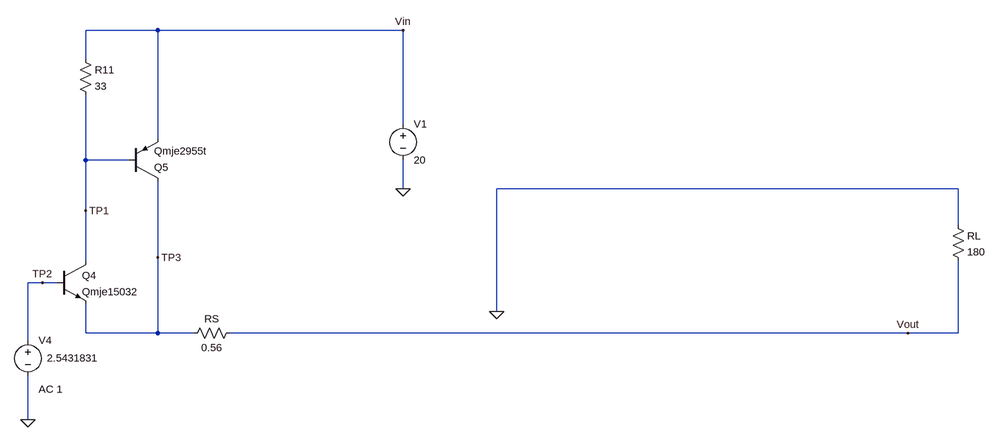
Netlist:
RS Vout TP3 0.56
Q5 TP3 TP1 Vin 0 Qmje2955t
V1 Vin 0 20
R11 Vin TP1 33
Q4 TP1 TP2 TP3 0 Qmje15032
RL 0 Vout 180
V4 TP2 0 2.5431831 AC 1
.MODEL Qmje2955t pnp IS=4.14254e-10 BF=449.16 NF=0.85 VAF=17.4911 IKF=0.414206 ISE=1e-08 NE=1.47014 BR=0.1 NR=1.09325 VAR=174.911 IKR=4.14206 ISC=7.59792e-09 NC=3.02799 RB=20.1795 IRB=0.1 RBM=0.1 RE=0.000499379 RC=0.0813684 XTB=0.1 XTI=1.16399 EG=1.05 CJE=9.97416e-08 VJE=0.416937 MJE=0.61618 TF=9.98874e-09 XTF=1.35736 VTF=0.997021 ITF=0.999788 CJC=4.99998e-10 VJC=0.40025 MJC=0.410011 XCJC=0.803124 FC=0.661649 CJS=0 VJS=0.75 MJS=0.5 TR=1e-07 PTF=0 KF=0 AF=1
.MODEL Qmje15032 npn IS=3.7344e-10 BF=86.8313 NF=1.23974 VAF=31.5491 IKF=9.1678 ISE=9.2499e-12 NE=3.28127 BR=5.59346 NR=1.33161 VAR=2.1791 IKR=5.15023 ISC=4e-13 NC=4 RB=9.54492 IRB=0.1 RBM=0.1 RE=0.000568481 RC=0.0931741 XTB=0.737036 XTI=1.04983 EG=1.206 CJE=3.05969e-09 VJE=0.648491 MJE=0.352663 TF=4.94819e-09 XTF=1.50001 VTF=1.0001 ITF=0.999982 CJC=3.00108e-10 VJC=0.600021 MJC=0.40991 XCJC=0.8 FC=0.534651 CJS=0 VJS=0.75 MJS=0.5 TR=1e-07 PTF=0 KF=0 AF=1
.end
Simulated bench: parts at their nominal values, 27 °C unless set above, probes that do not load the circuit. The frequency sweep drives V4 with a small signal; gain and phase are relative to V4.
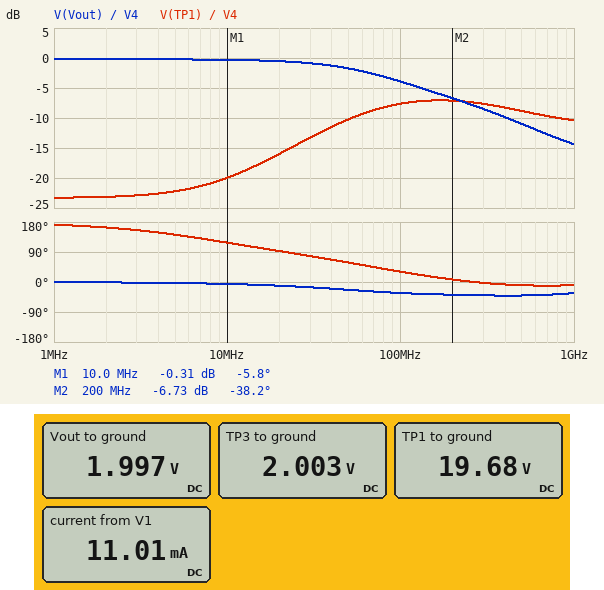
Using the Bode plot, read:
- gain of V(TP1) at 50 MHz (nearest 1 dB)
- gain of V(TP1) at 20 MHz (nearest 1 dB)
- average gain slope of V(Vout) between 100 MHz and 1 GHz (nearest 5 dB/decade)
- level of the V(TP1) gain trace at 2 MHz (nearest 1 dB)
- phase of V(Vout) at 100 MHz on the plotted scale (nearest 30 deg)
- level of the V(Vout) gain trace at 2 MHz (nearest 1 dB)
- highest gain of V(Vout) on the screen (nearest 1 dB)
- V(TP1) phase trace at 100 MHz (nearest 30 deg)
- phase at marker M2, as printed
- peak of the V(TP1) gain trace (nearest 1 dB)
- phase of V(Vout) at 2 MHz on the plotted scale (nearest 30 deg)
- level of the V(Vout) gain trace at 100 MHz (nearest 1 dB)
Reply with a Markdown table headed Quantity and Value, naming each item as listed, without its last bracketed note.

| Quantity | Value |
|---|---|
| gain of V(TP1) at 50 MHz | -10 dB |
| gain of V(TP1) at 20 MHz | -16 dB |
| average gain slope of V(Vout) between 100 MHz and 1 GHz | -10 dB/decade |
| level of the V(TP1) gain trace at 2 MHz | -23 dB |
| phase of V(Vout) at 100 MHz on the plotted scale | -30 deg |
| level of the V(Vout) gain trace at 2 MHz | 0 dB |
| highest gain of V(Vout) on the screen | 0 dB |
| V(TP1) phase trace at 100 MHz | 30 deg |
| phase at marker M2, as printed | -38.2 deg |
| peak of the V(TP1) gain trace | -7 dB |
| phase of V(Vout) at 2 MHz on the plotted scale | 0 deg |
| level of the V(Vout) gain trace at 100 MHz | -4 dB |
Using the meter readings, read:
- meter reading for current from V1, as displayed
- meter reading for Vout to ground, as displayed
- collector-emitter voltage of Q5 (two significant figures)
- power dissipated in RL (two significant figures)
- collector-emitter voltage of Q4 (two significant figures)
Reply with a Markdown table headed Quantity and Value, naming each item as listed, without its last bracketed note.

| Quantity | Value |
|---|---|
| meter reading for current from V1, as displayed | 11.01 mA |
| meter reading for Vout to ground, as displayed | 1.997 V |
| collector-emitter voltage of Q5 | -18 V |
| power dissipated in RL | 22 mW |
| collector-emitter voltage of Q4 | 18 V |
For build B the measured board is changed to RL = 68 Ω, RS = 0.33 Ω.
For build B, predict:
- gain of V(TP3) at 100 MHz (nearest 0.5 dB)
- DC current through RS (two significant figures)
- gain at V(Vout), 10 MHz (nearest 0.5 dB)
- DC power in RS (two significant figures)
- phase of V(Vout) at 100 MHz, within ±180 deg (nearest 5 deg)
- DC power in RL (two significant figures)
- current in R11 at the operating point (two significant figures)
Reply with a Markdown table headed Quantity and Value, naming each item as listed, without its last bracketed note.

| Quantity | Value |
|---|---|
| gain of V(TP3) at 100 MHz | -4.5 dB |
| DC current through RS | 29 mA |
| gain at V(Vout), 10 MHz | -1.0 dB |
| DC power in RS | 280 µW |
| phase of V(Vout) at 100 MHz, within ±180 deg | -30 deg |
| DC power in RL | 58 mW |
| current in R11 at the operating point | 11 mA |
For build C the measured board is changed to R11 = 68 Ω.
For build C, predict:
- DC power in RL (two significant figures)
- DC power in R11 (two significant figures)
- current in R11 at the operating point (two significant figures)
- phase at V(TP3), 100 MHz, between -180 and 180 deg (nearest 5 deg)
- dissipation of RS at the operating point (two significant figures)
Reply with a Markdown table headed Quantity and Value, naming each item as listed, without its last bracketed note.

| Quantity | Value |
|---|---|
| DC power in RL | 23 mW |
| DC power in R11 | 1.8 mW |
| current in R11 at the operating point | 5.1 mA |
| phase at V(TP3), 100 MHz, between -180 and 180 deg | -30 deg |
| dissipation of RS at the operating point | 70 µW |
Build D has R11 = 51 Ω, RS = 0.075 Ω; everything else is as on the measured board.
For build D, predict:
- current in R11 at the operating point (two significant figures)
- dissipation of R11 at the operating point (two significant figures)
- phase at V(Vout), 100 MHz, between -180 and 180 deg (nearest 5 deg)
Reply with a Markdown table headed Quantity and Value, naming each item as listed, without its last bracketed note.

| Quantity | Value |
|---|---|
| current in R11 at the operating point | 6.7 mA |
| dissipation of R11 at the operating point | 2.3 mW |
| phase at V(Vout), 100 MHz, between -180 and 180 deg | -30 deg |
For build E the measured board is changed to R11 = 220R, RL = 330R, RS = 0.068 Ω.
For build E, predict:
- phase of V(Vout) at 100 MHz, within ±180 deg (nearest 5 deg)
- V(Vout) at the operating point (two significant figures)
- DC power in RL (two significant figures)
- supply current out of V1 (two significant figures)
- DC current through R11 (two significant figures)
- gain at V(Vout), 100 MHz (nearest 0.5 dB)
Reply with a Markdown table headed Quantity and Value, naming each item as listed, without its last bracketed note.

| Quantity | Value |
|---|---|
| phase of V(Vout) at 100 MHz, within ±180 deg | -30 deg |
| V(Vout) at the operating point | 2.1 V |
| DC power in RL | 13 mW |
| supply current out of V1 | 6.2 mA |
| DC current through R11 | 1.6 mA |
| gain at V(Vout), 100 MHz | -3.5 dB |
